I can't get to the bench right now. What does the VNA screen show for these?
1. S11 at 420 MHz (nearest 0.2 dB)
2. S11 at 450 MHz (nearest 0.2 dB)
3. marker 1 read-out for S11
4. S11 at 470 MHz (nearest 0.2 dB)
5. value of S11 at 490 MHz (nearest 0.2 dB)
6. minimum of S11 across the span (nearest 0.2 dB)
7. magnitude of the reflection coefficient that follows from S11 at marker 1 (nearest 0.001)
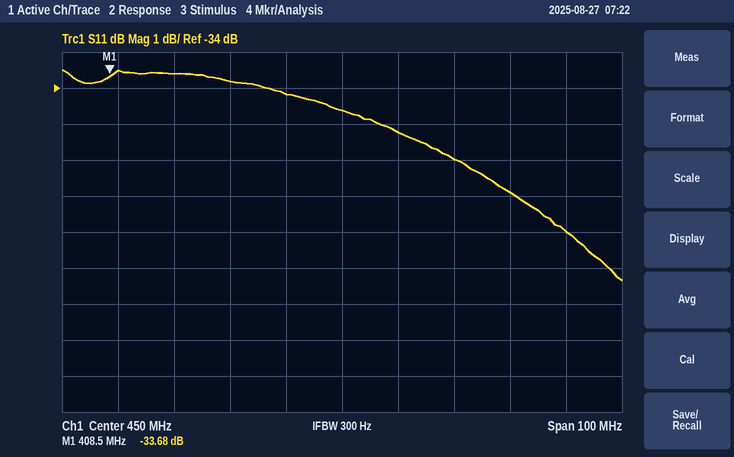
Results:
-33.6 dB
-34.6 dB
-33.68 dB
-36.0 dB
-38.0 dB
-39.4 dB
0.021
